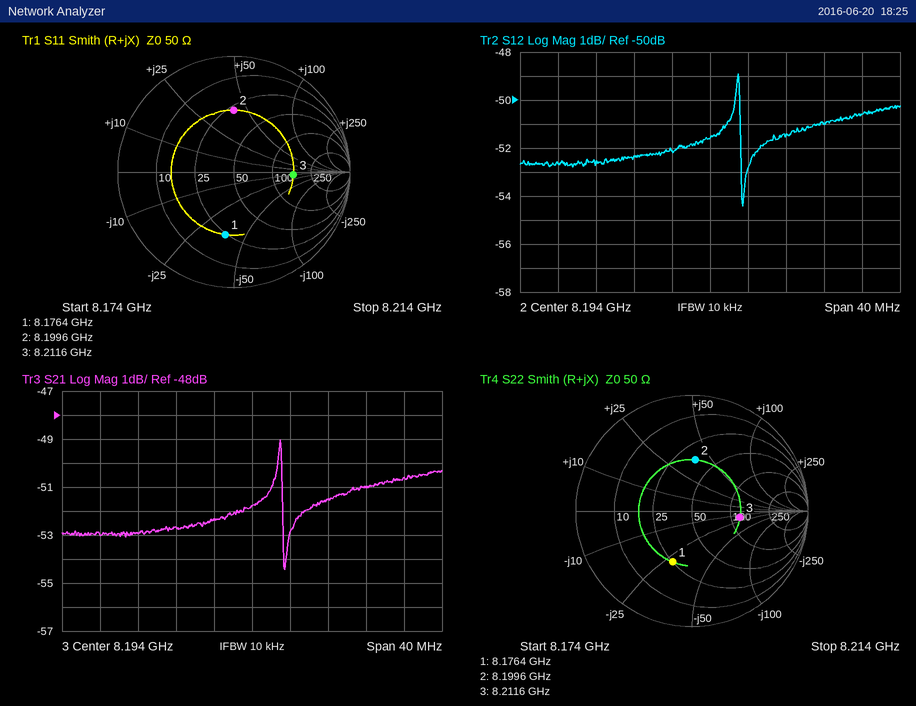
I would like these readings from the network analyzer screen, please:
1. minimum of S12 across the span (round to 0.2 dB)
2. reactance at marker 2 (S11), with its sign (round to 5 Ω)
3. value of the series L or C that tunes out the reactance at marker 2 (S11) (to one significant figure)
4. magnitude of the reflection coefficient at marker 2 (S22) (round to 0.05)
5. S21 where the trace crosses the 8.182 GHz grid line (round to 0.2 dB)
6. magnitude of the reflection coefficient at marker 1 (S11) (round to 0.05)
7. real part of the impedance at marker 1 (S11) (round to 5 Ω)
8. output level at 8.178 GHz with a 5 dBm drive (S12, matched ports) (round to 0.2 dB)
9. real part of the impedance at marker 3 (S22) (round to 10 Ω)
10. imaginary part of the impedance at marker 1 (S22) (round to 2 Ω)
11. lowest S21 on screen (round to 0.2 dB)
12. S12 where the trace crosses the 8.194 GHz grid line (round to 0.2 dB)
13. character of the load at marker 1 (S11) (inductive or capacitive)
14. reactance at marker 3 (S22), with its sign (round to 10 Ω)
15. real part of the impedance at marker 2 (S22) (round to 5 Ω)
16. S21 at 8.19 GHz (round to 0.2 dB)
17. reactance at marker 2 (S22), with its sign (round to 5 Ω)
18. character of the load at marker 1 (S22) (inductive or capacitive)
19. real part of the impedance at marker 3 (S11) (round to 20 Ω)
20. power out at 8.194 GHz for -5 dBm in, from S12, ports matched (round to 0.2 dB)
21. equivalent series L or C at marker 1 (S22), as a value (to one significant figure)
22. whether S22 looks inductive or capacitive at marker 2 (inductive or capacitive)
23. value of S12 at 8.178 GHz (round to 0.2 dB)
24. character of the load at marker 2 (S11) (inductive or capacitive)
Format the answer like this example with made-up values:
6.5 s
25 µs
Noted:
-54.4 dB
+40 Ω
500 fF
0.45
-53.0 dB
0.55
25 Ω
-47.6 dBm
120 Ω
-28 Ω
-54.4 dB
-51.6 dB
capacitive
-20 Ω
35 Ω
-52.4 dB
+40 Ω
capacitive
160 Ω
-56.6 dBm
700 fF
inductive
-52.6 dB
inductive
